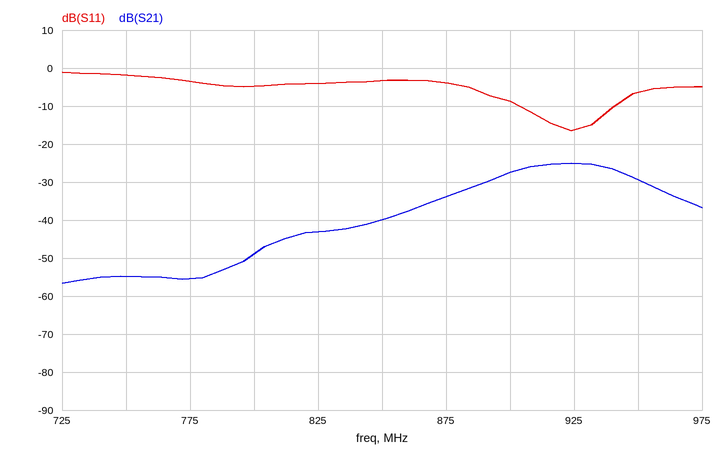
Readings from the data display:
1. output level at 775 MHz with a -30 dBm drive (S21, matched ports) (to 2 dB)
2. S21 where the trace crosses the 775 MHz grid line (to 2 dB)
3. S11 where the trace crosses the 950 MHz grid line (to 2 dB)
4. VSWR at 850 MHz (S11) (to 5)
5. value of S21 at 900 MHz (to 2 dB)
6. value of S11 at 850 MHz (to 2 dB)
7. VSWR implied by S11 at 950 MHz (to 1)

-86 dBm
-56 dB
-6 dB
5
-28 dB
-4 dB
3
